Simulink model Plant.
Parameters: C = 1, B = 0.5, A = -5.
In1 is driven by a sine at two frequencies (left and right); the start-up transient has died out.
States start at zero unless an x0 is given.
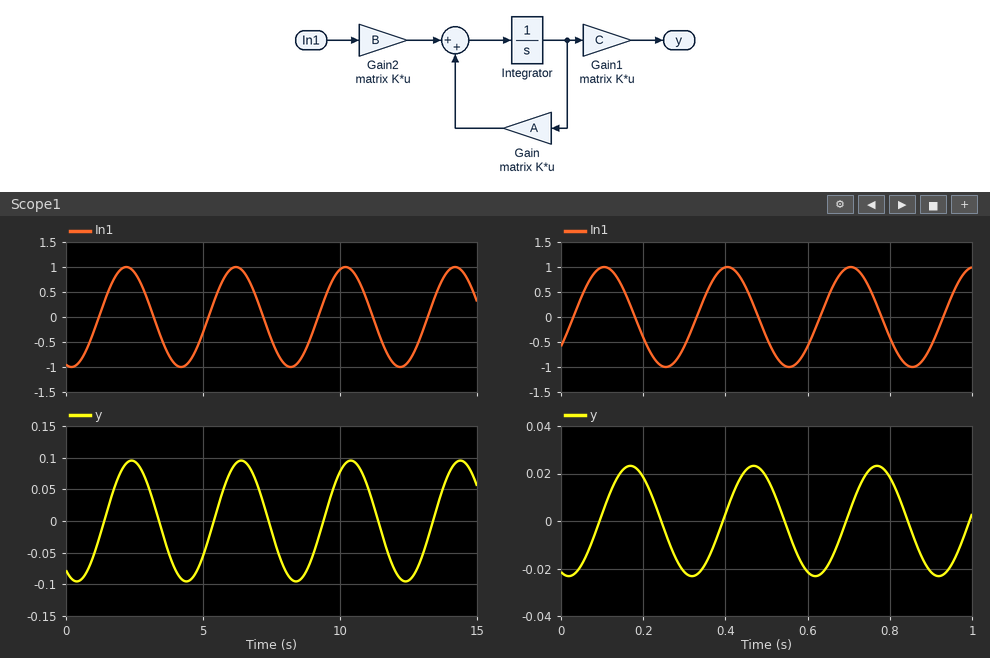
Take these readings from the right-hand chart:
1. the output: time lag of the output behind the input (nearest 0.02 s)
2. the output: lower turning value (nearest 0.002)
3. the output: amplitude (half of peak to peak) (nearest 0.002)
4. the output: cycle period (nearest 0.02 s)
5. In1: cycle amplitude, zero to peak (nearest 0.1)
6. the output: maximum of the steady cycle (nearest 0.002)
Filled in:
0.06 s
-0.024
0.024
0.30 s
1.0
0.024
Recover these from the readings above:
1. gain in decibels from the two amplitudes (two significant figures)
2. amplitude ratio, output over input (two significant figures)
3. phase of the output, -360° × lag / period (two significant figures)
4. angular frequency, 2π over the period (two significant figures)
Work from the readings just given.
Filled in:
-32 dB
0.024
-72°
21 rad/s
